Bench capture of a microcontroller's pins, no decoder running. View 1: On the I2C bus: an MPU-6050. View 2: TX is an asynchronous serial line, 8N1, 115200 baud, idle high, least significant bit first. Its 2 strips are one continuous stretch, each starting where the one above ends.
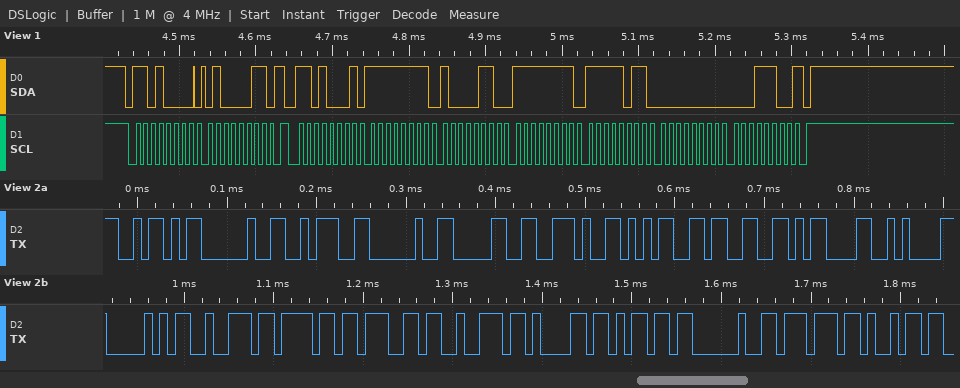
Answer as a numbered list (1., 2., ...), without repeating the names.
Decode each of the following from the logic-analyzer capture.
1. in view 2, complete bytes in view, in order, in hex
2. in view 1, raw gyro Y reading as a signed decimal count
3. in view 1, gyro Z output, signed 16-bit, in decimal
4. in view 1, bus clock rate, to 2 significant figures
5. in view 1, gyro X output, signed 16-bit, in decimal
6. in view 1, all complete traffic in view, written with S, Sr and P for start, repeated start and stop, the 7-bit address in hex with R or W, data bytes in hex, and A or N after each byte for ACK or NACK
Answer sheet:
1. 5A 20 3A 20 30 2E 35 33 0D 0A 50 72 6F 67 72 61 6D 20 77 69
2. -5
3. 28
4. 100 kHz
5. -122
6. S 68W A 43 A Sr 68R A FF A 86 A FF A FB A 00 A 1C N P
